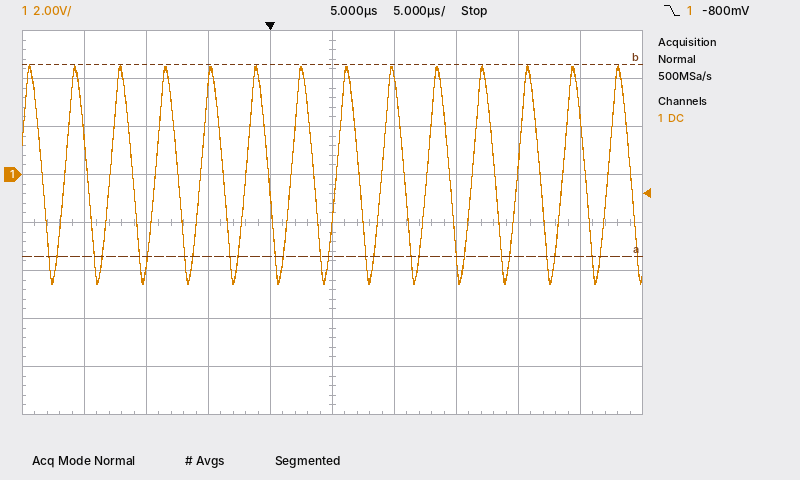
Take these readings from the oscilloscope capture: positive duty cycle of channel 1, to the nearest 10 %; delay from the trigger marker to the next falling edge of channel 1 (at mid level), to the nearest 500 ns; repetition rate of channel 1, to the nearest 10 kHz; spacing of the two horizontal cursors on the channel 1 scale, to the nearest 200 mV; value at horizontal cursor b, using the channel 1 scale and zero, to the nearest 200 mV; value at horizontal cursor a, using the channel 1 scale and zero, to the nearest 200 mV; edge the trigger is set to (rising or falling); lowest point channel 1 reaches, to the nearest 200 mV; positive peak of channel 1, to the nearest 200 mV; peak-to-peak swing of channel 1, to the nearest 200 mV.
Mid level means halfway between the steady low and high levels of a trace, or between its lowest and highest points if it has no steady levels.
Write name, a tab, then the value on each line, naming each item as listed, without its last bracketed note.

positive duty cycle of channel 1, to the nearest 10 %	50 %
delay from the trigger marker to the next falling edge of channel 1 (at mid level), to the nearest 500 ns	3.5 µs
repetition rate of channel 1, to the nearest 10 kHz	270 kHz
spacing of the two horizontal cursors on the channel 1 scale, to the nearest 200 mV	8.0 V
value at horizontal cursor b, using the channel 1 scale and zero, to the nearest 200 mV	4.6 V
value at horizontal cursor a, using the channel 1 scale and zero, to the nearest 200 mV	-3.4 V
edge the trigger is set to	falling
lowest point channel 1 reaches, to the nearest 200 mV	-4.6 V
positive peak of channel 1, to the nearest 200 mV	4.6 V
peak-to-peak swing of channel 1, to the nearest 200 mV	9.2 V
